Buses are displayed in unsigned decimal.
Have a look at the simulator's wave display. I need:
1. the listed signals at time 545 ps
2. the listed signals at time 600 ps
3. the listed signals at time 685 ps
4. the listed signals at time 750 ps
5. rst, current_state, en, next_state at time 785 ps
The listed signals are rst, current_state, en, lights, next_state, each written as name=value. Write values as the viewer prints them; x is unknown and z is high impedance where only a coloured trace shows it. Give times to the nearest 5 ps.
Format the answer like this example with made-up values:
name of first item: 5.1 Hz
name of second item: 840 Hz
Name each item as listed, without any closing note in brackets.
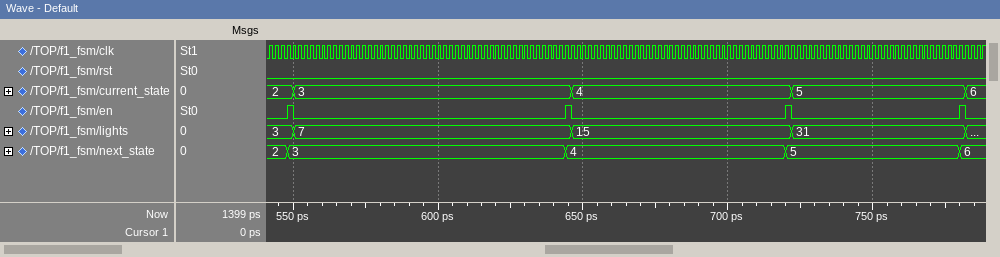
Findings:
the listed signals at time 545 ps: rst=0, current_state=2, en=0, lights=3, next_state=2
the listed signals at time 600 ps: rst=0, current_state=3, en=0, lights=7, next_state=3
the listed signals at time 685 ps: rst=0, current_state=4, en=0, lights=15, next_state=4
the listed signals at time 750 ps: rst=0, current_state=5, en=0, lights=31, next_state=5
rst, current_state, en, next_state at time 785 ps: rst=0, current_state=6, en=0, next_state=6
